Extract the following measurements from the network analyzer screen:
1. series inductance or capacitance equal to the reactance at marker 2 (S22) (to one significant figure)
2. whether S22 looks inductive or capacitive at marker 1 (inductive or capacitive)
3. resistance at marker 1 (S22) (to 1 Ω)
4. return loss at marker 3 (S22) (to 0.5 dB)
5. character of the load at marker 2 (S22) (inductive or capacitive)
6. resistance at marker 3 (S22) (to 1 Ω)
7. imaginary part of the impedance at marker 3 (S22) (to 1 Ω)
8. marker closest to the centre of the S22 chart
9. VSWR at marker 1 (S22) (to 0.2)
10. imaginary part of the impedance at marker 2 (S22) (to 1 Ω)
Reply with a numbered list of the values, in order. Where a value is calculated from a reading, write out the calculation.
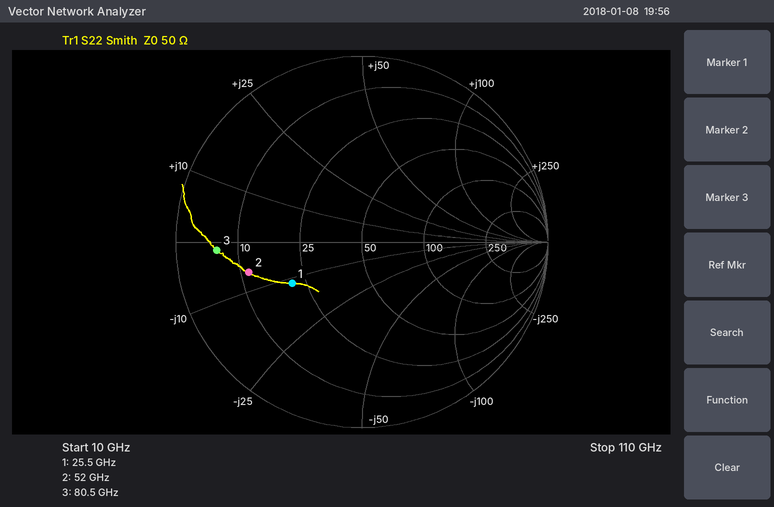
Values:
1. C = 1/(2π × 52 GHz × 6 Ω) ≈ 510 fF, so 500 fF to one significant figure
2. capacitive
3. 21 Ω
4. 2.0 dB
5. capacitive
6. 6 Ω
7. -1 Ω
8. marker 1
9. 2.6
10. -6 Ω
